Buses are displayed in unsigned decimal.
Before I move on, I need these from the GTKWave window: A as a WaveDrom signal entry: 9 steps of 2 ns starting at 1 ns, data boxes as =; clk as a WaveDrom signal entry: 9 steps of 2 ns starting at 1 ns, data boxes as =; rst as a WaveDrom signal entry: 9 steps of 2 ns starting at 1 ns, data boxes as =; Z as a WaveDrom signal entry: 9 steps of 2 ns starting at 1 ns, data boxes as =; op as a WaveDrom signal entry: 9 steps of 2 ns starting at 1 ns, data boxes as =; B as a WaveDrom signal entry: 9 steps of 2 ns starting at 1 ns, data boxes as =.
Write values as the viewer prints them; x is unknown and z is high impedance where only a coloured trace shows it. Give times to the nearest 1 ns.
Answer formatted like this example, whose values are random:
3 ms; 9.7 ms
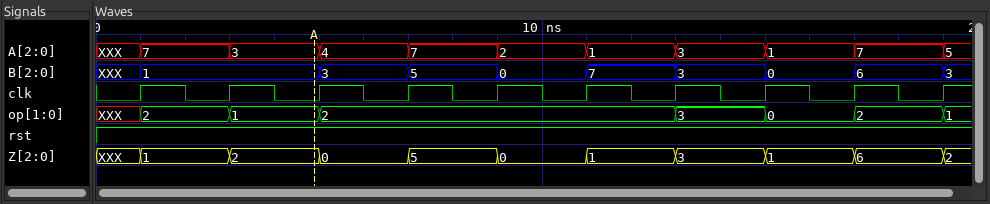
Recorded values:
{name: 'A', wave: '=========', data: '7 3 4 7 2 1 3 1 7'}; {name: 'clk', wave: 'p........'}; {name: 'rst', wave: '1........'}; {name: 'Z', wave: '=========', data: '1 2 0 5 0 1 3 1 6'}; {name: 'op', wave: '===...===', data: '2 1 2 3 0 2'}; {name: 'B', wave: '=.=======', data: '1 3 5 0 7 3 0 6'}
